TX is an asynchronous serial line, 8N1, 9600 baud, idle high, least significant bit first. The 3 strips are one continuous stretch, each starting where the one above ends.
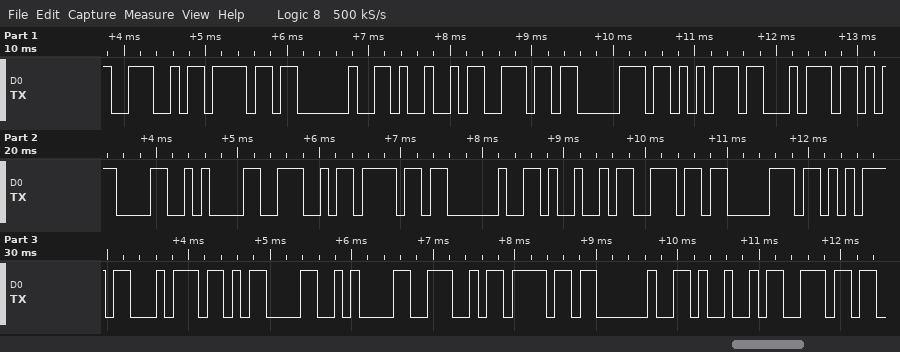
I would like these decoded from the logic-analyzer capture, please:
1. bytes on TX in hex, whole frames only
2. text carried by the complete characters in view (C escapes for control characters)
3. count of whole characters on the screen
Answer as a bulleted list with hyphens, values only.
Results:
- 4E 6F 20 49 6E 70 75 74 0D 0A 4E 6F 20 49 6E 70 75 74 0D 0A 4E 6F 20 49 6E
- "No Input\r\nNo Input\r\nNo In"
- 25
